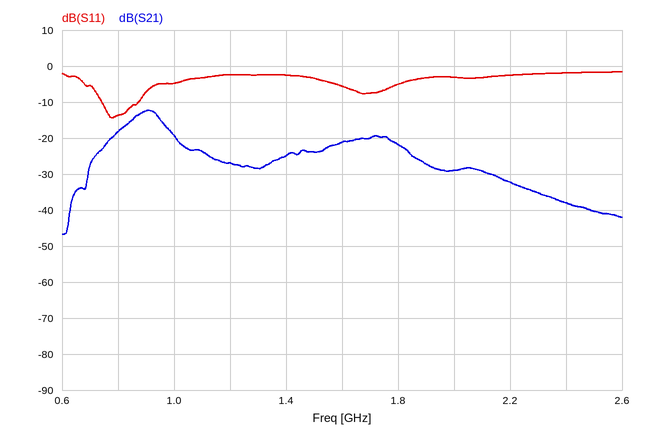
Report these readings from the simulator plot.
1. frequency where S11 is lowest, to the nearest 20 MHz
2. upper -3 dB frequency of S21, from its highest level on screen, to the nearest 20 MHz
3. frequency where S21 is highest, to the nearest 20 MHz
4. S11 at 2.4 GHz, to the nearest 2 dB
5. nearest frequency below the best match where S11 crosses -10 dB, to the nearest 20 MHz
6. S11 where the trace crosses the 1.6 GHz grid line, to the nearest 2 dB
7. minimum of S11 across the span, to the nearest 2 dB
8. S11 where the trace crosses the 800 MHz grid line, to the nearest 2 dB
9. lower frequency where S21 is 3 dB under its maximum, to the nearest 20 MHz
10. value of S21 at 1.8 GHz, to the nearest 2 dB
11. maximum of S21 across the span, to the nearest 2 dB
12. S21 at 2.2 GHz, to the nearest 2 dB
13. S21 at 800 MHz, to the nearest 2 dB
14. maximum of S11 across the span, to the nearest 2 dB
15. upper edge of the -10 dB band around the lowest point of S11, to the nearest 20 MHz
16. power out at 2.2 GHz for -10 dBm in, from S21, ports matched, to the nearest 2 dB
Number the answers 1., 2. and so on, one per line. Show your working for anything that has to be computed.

1. 780 MHz
2. 960 MHz
3. 900 MHz
4. -2 dB
5. 740 MHz
6. -6 dB
7. -14 dB
8. -14 dB
9. 840 MHz
10. -22 dB
11. -12 dB
12. -32 dB
13. -18 dB
14. -2 dB
15. 880 MHz
16. -10 dBm + (-32 dB) = -42 dBm
